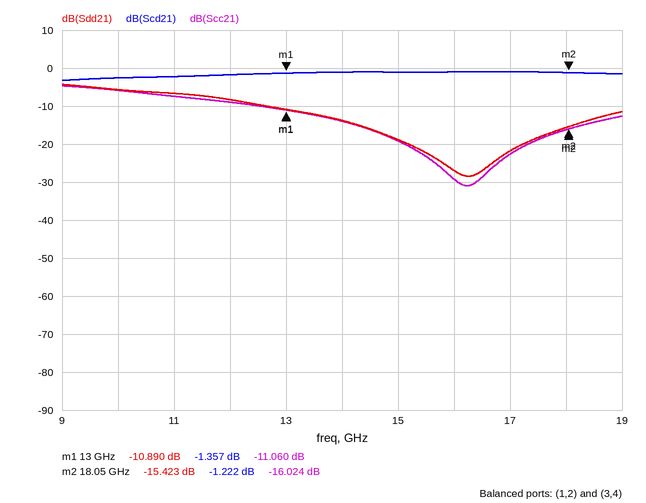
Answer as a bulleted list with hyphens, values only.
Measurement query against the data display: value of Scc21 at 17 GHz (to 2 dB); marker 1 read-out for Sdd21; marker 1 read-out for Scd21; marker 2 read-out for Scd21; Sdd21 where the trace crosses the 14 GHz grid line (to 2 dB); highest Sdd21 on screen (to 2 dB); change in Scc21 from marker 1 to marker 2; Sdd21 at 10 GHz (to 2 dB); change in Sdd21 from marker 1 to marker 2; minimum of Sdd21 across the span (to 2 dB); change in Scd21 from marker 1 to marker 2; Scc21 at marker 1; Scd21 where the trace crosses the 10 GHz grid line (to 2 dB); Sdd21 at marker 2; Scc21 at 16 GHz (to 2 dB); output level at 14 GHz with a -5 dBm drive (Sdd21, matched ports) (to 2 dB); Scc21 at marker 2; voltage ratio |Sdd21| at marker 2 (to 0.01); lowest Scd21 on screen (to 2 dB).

- -22 dB
- -10.890 dB
- -1.357 dB
- -1.222 dB
- -14 dB
- -4 dB
- -4.964 dB
- -6 dB
- -4.533 dB
- -28 dB
- 0.135 dB
- -11.060 dB
- -2 dB
- -15.423 dB
- -30 dB
- -18 dBm
- -16.024 dB
- 0.17
- -4 dB
